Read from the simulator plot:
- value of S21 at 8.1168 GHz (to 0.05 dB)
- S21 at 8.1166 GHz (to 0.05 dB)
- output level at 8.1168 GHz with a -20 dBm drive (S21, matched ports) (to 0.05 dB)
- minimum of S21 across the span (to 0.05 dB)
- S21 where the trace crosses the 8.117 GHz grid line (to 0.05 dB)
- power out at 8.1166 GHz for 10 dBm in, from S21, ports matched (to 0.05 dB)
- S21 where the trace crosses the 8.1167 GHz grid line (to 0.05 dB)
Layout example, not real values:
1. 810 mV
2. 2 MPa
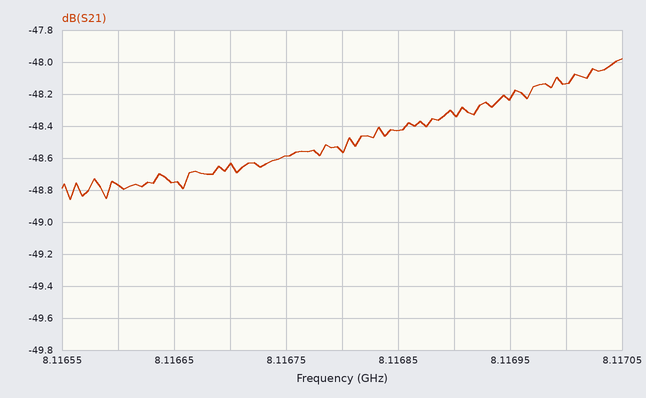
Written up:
1. -48.55 dB
2. -48.75 dB
3. -68.55 dBm
4. -48.85 dB
5. -48.15 dB
6. -38.75 dBm
7. -48.65 dB
